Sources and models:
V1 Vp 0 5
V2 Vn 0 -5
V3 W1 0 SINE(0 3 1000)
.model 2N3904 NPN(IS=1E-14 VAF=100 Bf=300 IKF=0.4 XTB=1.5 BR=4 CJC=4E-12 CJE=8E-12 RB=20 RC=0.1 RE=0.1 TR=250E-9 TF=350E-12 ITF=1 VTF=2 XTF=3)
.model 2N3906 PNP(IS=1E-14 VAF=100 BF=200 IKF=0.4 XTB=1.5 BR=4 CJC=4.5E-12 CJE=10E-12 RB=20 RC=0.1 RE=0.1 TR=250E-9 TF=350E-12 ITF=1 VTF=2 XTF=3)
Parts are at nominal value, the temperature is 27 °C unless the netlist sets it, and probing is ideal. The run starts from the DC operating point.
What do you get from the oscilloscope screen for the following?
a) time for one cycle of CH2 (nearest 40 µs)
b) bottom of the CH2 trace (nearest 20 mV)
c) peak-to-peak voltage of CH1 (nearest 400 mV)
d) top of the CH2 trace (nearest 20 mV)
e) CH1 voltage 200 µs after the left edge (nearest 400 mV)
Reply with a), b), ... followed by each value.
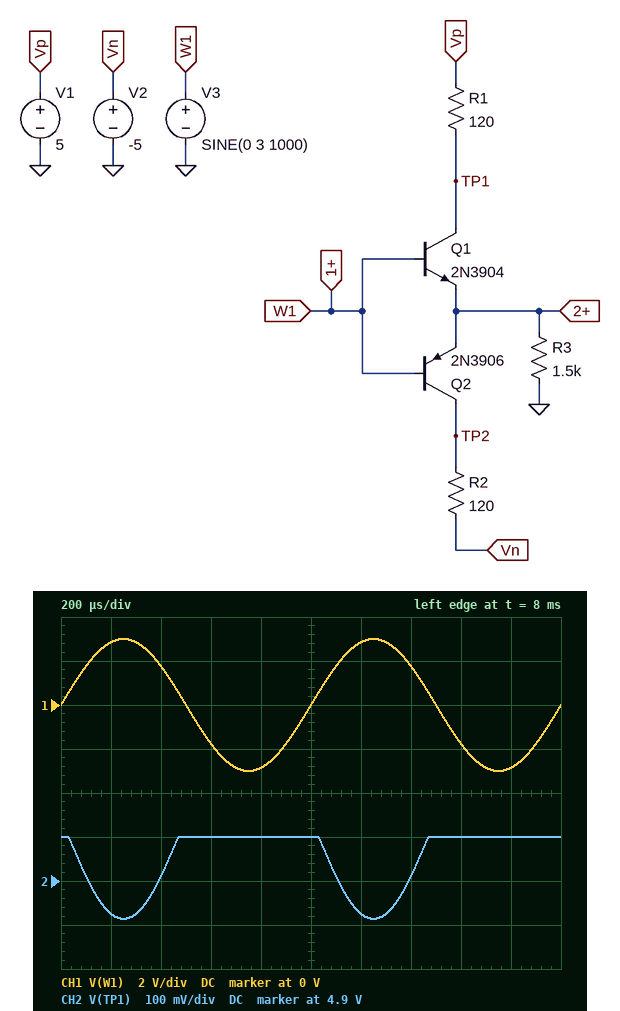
a) 1.00 ms
b) 4.82 V
c) 6.0 V
d) 5.00 V
e) 2.8 V
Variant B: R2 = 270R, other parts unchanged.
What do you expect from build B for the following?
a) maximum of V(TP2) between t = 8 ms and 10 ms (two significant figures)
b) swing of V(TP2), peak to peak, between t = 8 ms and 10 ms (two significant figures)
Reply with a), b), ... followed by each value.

a) -4.6 V
b) 420 mV
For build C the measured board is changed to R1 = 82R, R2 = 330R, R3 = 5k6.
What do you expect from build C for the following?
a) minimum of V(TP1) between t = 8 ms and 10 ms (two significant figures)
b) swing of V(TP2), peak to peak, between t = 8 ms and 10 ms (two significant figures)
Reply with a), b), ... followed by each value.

a) 5.0 V
b) 140 mV
